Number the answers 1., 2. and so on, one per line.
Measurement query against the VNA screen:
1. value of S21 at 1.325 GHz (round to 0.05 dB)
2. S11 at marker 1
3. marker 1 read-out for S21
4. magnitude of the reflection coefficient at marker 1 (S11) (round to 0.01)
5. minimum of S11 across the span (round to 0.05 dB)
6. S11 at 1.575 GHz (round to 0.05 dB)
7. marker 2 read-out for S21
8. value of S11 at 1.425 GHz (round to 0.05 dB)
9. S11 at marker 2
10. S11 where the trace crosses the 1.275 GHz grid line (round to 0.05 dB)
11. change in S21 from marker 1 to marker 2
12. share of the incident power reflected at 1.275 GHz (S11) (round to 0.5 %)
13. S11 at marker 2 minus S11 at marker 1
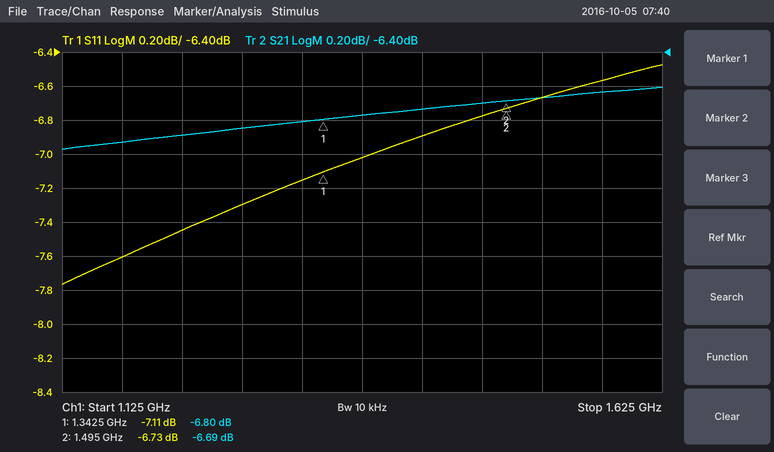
1. -6.80 dB
2. -7.11 dB
3. -6.80 dB
4. 0.44
5. -7.75 dB
6. -6.55 dB
7. -6.69 dB
8. -6.90 dB
9. -6.73 dB
10. -7.30 dB
11. 0.11 dB
12. 18.5 %
13. 0.38 dB
